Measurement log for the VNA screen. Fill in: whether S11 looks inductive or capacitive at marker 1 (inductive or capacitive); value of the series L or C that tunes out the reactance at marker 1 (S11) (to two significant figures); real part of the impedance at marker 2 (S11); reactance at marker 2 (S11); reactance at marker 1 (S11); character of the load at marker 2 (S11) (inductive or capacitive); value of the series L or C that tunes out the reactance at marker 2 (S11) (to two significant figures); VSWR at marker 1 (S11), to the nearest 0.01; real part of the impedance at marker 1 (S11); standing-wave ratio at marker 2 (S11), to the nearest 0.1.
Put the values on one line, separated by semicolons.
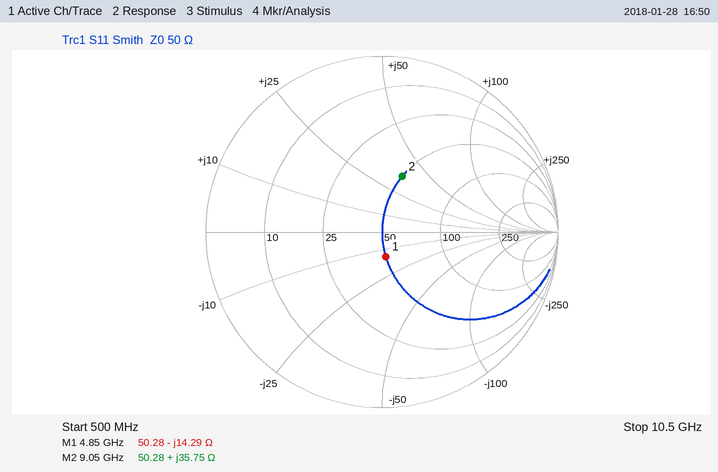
capacitive; 470 pH; 50.28 Ω; +35.75 Ω; -14.29 Ω; inductive; 490 fF; 1.33; 50.28 Ω; 2.0
